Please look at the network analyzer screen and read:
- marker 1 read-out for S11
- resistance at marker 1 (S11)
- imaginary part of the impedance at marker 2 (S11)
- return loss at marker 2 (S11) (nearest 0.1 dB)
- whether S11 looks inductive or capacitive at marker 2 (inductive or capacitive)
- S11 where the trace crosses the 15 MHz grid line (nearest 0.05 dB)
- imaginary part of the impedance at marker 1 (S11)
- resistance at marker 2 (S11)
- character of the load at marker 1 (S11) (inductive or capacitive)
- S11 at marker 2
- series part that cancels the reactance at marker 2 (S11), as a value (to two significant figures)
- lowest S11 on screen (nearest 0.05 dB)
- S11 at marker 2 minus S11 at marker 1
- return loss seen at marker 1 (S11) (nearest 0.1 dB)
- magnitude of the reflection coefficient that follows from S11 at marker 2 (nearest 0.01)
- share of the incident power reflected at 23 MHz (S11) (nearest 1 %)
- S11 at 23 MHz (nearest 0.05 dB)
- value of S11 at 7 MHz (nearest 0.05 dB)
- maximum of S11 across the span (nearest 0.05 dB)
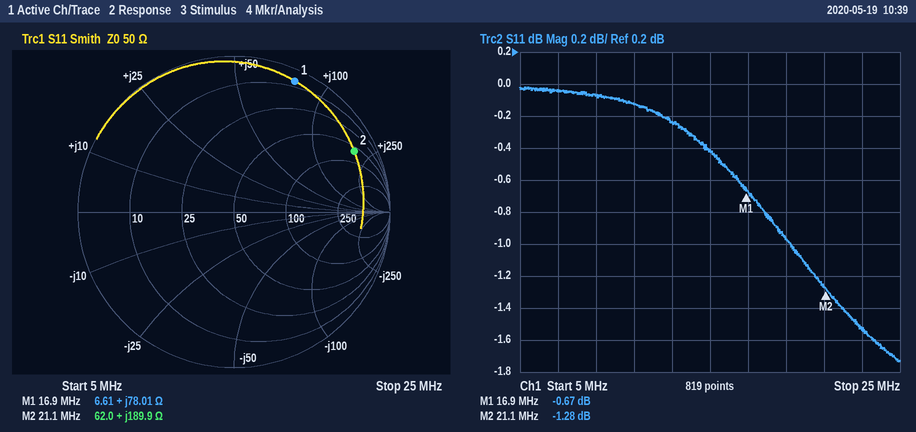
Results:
-0.67 dB
6.61 Ω
+189.9 Ω
1.3 dB
inductive
-0.40 dB
+78.01 Ω
62.0 Ω
inductive
-1.28 dB
40 pF
-1.75 dB
-0.61 dB
0.7 dB
0.86
70 %
-1.55 dB
-0.05 dB
0.00 dB
